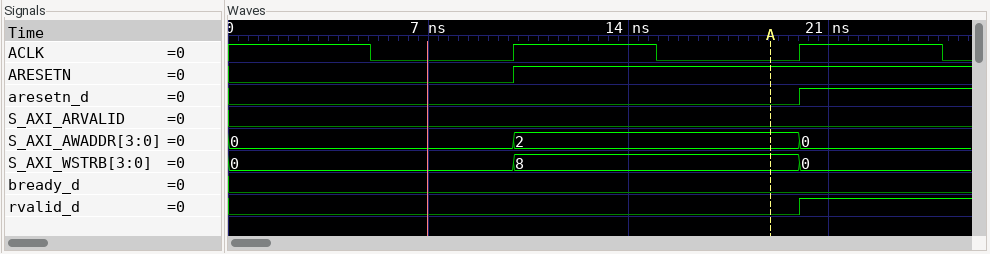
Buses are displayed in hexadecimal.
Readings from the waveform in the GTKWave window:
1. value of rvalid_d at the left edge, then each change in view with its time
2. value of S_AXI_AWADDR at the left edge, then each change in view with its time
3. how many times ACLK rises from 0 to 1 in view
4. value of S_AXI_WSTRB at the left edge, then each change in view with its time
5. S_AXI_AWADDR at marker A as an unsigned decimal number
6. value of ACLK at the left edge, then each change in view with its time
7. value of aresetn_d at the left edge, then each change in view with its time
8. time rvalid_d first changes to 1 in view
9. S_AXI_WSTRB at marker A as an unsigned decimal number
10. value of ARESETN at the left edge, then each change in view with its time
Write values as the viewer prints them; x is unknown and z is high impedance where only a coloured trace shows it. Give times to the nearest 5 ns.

0, 1 at 20 ns
0, 2 at 10 ns, 0 at 20 ns
2
0, 8 at 10 ns, 0 at 20 ns
2
1, 0 at 5 ns, 1 at 10 ns, 0 at 15 ns, 1 at 20 ns, 0 at 25 ns
0, 1 at 20 ns
20 ns
8
0, 1 at 10 ns
